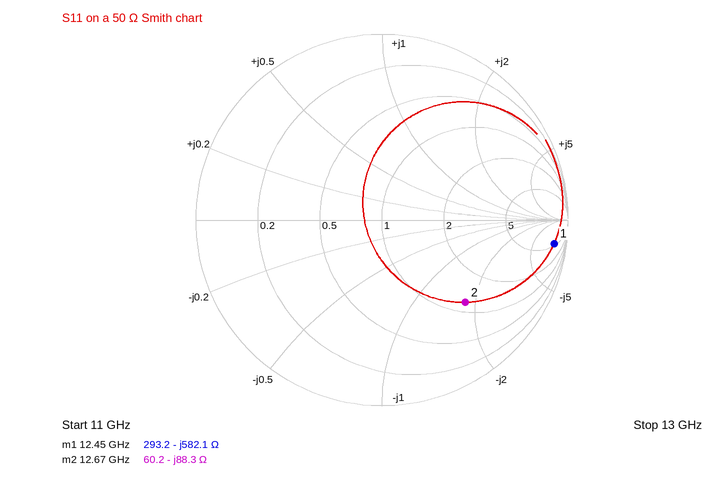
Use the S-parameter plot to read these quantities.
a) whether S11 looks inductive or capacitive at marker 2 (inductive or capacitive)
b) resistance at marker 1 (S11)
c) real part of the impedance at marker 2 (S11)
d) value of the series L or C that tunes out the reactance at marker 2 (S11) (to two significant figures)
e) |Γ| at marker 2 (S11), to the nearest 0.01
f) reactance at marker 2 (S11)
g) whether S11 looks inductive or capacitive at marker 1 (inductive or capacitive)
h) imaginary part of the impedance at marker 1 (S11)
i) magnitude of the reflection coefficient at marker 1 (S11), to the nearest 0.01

capacitive
293.2 Ω
60.2 Ω
1.1 nH
0.63
-88.3 Ω
capacitive
-582.1 Ω
0.93
